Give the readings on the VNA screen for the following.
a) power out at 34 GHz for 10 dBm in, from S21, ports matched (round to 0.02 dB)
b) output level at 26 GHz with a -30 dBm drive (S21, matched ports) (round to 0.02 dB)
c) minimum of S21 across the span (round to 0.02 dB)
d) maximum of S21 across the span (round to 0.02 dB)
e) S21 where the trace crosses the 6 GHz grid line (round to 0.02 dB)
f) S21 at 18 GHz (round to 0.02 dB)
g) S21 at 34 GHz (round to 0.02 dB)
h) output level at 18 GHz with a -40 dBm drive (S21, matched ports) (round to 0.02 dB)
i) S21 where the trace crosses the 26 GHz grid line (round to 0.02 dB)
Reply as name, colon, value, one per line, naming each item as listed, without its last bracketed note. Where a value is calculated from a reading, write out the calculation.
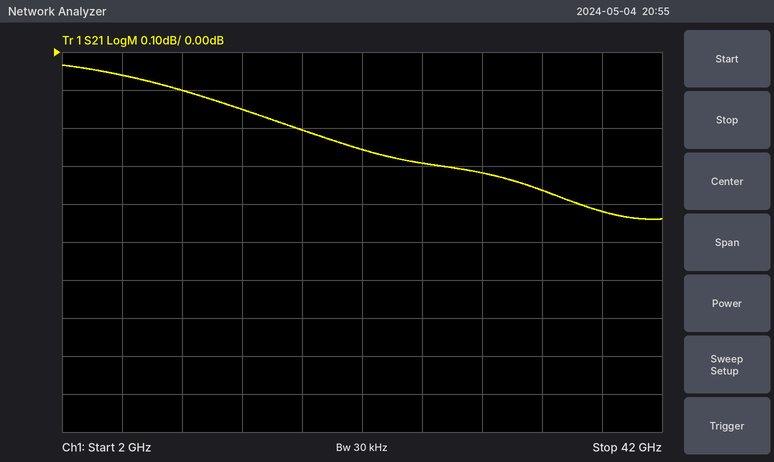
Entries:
power out at 34 GHz for 10 dBm in, from S21, ports matched: 10 dBm + (-0.36 dB) = 9.64 dBm
output level at 26 GHz with a -30 dBm drive (S21, matched ports): -30 dBm + (-0.30 dB) = -30.30 dBm
minimum of S21 across the span: -0.44 dB
maximum of S21 across the span: -0.04 dB
S21 where the trace crosses the 6 GHz grid line: -0.06 dB
S21 at 18 GHz: -0.20 dB
S21 at 34 GHz: -0.36 dB
output level at 18 GHz with a -40 dBm drive (S21, matched ports): -40 dBm + (-0.20 dB) = -40.20 dBm
S21 where the trace crosses the 26 GHz grid line: -0.30 dB
